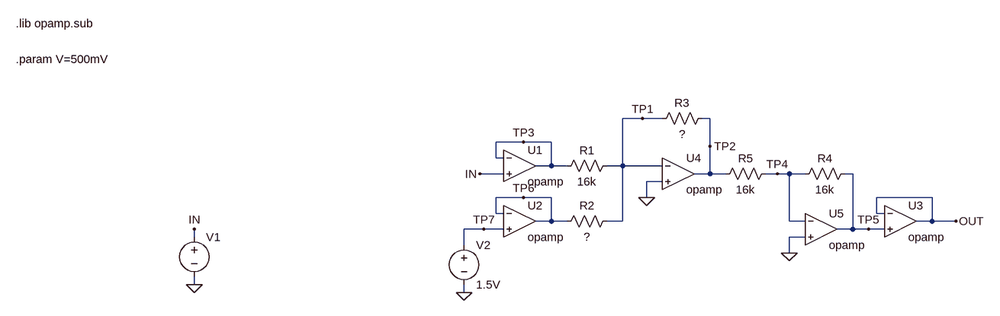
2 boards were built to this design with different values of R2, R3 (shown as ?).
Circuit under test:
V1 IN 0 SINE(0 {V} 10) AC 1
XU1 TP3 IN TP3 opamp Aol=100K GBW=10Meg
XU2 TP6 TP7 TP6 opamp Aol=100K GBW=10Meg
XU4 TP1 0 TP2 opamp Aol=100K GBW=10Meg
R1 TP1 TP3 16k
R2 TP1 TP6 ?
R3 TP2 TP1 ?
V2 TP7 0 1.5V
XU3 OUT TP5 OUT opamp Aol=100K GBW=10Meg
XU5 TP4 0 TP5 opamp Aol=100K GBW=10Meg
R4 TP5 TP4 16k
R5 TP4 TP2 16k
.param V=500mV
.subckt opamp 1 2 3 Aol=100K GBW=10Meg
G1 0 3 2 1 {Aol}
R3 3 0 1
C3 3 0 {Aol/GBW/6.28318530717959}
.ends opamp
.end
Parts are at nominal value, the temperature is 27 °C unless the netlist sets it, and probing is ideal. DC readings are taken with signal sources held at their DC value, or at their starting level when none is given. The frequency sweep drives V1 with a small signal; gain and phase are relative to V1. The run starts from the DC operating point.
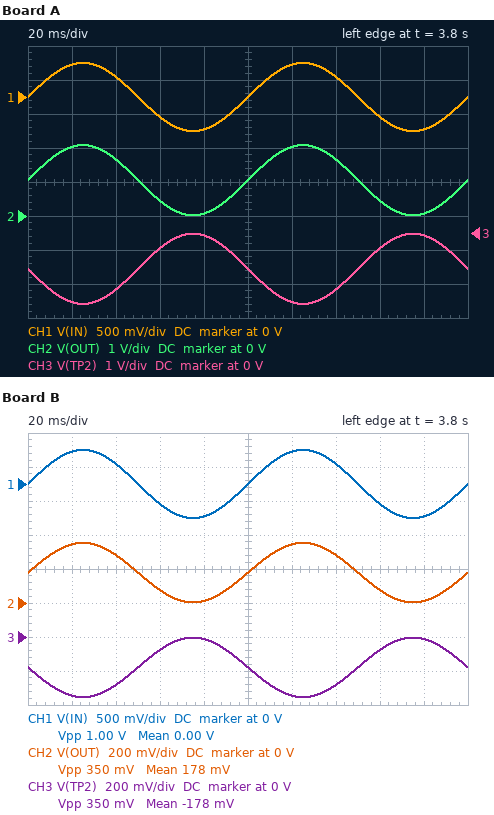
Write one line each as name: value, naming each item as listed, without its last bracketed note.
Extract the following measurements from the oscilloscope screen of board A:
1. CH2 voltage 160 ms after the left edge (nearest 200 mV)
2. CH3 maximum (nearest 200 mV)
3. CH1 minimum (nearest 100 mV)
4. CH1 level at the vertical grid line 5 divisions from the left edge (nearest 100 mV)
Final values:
CH2 voltage 160 ms after the left edge: 400 mV
CH3 maximum: 0 V
CH1 minimum: -500 mV
CH1 level at the vertical grid line 5 divisions from the left edge: 0 V
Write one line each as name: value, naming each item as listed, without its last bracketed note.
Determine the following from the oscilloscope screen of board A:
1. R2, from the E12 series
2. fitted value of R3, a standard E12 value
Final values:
R2, from the E12 series: 47 kΩ
fitted value of R3, a standard E12 value: 33 kΩ
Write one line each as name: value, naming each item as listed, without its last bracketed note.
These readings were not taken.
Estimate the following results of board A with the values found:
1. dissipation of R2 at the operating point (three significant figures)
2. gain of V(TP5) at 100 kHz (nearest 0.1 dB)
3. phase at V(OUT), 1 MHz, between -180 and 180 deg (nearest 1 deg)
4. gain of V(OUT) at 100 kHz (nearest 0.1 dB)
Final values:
dissipation of R2 at the operating point: 47.9 µW
gain of V(TP5) at 100 kHz: 6.3 dB
phase at V(OUT), 1 MHz, between -180 and 180 deg: -43 deg
gain of V(OUT) at 100 kHz: 6.3 dB
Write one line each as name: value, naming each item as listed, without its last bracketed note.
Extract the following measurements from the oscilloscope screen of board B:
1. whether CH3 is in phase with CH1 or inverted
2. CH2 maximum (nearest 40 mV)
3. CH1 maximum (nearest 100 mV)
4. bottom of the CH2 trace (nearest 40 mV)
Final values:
whether CH3 is in phase with CH1 or inverted: inverted
CH2 maximum: 360 mV
CH1 maximum: 500 mV
bottom of the CH2 trace: 0 V
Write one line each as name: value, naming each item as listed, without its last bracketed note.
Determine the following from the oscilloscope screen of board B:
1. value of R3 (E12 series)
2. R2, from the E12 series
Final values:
value of R3: 5.6 kΩ
R2, from the E12 series: 47 kΩ
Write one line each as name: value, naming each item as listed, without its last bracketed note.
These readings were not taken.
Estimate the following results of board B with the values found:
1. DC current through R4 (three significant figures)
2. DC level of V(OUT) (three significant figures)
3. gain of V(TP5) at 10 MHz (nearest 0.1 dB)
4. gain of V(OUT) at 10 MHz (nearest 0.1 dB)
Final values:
DC current through R4: 11.2 µA
DC level of V(OUT): 179 mV
gain of V(TP5) at 10 MHz: -24.1 dB
gain of V(OUT) at 10 MHz: -27.1 dB
